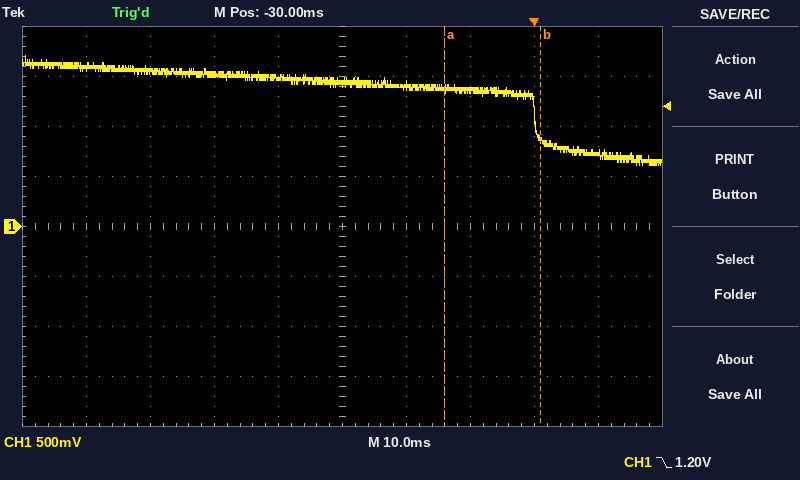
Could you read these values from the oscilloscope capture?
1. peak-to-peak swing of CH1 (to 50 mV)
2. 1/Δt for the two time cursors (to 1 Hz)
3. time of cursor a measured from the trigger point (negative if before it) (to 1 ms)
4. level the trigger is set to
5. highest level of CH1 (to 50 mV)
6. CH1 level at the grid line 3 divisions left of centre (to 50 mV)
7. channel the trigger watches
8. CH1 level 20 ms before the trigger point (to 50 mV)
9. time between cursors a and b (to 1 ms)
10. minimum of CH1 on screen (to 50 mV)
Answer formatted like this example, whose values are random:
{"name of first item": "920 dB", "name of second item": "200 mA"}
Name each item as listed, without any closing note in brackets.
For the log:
{"peak-to-peak swing of CH1": "1.10 V", "1/Δt for the two time cursors": "67 Hz", "time of cursor a measured from the trigger point (negative if before it)": "-14 ms", "level the trigger is set to": "1.20 V", "highest level of CH1": "1.70 V", "CH1 level at the grid line 3 divisions left of centre": "1.55 V", "channel the trigger watches": "CH1", "CH1 level 20 ms before the trigger point": "1.40 V", "time between cursors a and b": "15 ms", "minimum of CH1 on screen": "600 mV"}
